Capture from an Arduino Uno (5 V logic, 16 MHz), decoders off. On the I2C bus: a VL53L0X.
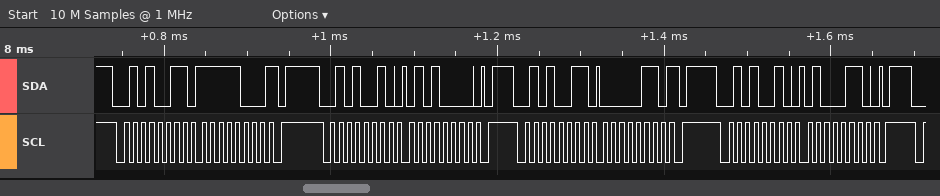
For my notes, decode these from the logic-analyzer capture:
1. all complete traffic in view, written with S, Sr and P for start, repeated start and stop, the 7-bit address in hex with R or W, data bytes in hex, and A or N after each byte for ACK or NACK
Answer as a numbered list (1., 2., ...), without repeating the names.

1. S 29R A F8 N P S 29W A 50 A P S 29R A 06 N P S 29W A 46 A P
